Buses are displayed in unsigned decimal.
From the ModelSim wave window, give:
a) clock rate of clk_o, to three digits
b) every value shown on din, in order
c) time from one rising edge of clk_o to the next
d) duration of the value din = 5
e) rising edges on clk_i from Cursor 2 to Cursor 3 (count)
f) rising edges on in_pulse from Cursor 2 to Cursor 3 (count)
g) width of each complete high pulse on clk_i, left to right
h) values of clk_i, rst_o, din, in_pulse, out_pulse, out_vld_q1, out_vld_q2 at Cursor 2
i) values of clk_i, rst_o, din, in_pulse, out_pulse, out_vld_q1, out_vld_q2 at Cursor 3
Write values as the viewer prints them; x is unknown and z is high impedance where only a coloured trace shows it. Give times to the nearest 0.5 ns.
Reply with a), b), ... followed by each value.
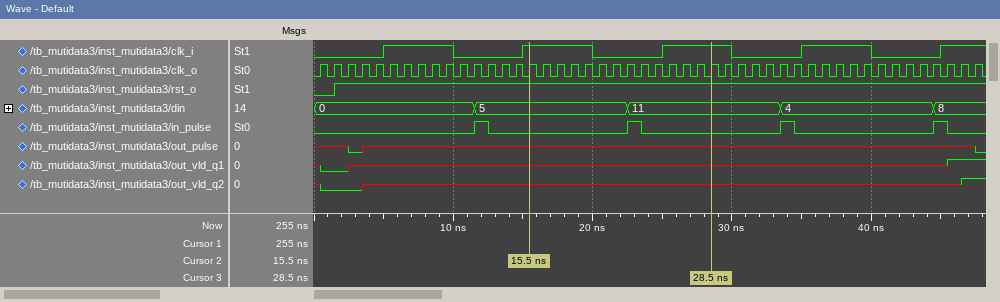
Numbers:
a) 1.00 GHz
b) 0, 5, 11, 4, 8
c) 1 ns
d) 11 ns
e) 1
f) 1
g) 5 ns, 5 ns, 5 ns, 5 ns
h) clk_i=1, rst_o=1, din=5, in_pulse=0, out_pulse=x, out_vld_q1=x, out_vld_q2=x
i) clk_i=1, rst_o=1, din=11, in_pulse=0, out_pulse=x, out_vld_q1=x, out_vld_q2=x
